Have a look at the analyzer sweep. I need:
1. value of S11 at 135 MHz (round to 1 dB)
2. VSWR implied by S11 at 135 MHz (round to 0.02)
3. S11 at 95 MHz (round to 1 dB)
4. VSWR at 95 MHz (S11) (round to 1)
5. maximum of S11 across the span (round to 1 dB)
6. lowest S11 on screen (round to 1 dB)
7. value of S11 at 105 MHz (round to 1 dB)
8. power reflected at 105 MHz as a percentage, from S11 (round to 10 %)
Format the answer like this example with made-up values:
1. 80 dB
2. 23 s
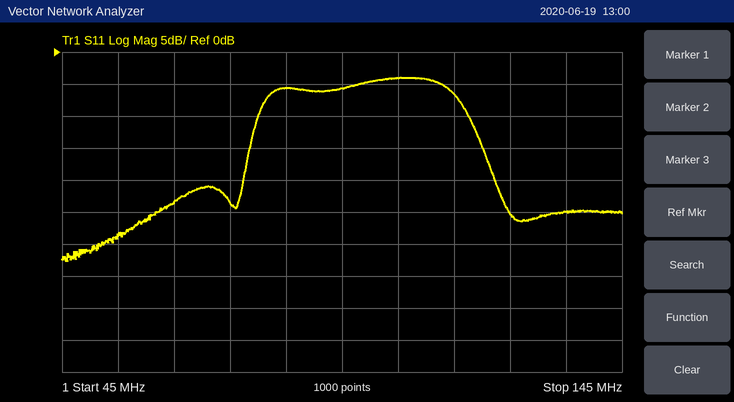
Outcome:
1. -25 dB
2. 1.12
3. -6 dB
4. 3
5. -4 dB
6. -33 dB
7. -4 dB
8. 40 %
